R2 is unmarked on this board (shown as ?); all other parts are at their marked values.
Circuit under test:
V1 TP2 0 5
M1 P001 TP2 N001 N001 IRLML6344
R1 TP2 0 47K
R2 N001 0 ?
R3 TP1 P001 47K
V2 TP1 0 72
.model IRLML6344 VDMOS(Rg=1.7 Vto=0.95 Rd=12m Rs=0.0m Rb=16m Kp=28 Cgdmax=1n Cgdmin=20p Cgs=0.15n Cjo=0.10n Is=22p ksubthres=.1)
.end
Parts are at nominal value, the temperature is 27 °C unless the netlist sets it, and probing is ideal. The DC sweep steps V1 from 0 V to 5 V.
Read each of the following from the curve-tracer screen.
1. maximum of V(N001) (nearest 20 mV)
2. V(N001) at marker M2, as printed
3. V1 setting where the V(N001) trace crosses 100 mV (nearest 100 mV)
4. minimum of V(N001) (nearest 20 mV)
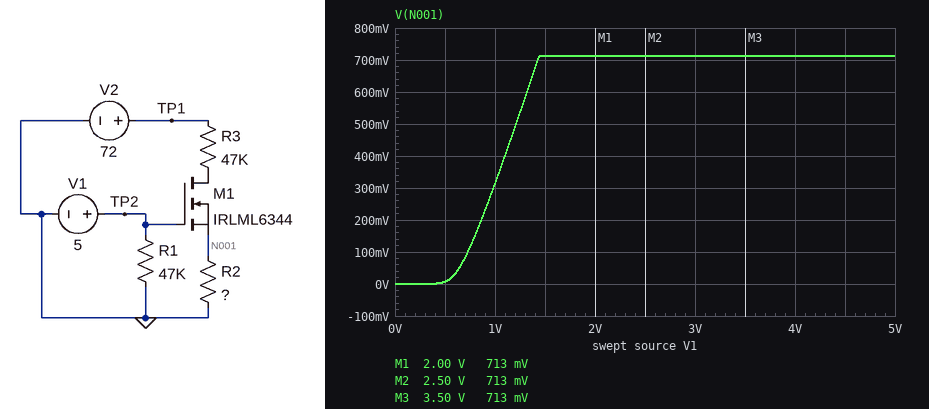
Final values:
720 mV
713 mV
700 mV
0 V
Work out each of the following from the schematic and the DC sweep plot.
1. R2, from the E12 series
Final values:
470 Ω
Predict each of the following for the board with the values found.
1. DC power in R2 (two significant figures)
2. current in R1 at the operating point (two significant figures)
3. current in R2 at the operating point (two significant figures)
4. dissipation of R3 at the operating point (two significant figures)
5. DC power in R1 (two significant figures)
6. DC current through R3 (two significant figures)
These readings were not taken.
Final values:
1.1 mW
110 µA
1.5 mA
110 mW
530 µW
1.5 mA
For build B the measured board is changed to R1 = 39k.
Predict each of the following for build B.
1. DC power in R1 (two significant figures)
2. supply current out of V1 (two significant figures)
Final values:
640 µW
130 µA
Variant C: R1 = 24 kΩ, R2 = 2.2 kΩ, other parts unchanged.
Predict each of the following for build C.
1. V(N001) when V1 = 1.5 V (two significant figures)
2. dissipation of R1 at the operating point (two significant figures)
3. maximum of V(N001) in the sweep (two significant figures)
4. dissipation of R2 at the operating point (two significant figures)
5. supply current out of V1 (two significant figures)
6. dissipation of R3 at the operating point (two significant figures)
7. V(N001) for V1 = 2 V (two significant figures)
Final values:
840 mV
1.0 mW
3.2 V
4.7 mW
210 µA
100 mW
1.3 V
